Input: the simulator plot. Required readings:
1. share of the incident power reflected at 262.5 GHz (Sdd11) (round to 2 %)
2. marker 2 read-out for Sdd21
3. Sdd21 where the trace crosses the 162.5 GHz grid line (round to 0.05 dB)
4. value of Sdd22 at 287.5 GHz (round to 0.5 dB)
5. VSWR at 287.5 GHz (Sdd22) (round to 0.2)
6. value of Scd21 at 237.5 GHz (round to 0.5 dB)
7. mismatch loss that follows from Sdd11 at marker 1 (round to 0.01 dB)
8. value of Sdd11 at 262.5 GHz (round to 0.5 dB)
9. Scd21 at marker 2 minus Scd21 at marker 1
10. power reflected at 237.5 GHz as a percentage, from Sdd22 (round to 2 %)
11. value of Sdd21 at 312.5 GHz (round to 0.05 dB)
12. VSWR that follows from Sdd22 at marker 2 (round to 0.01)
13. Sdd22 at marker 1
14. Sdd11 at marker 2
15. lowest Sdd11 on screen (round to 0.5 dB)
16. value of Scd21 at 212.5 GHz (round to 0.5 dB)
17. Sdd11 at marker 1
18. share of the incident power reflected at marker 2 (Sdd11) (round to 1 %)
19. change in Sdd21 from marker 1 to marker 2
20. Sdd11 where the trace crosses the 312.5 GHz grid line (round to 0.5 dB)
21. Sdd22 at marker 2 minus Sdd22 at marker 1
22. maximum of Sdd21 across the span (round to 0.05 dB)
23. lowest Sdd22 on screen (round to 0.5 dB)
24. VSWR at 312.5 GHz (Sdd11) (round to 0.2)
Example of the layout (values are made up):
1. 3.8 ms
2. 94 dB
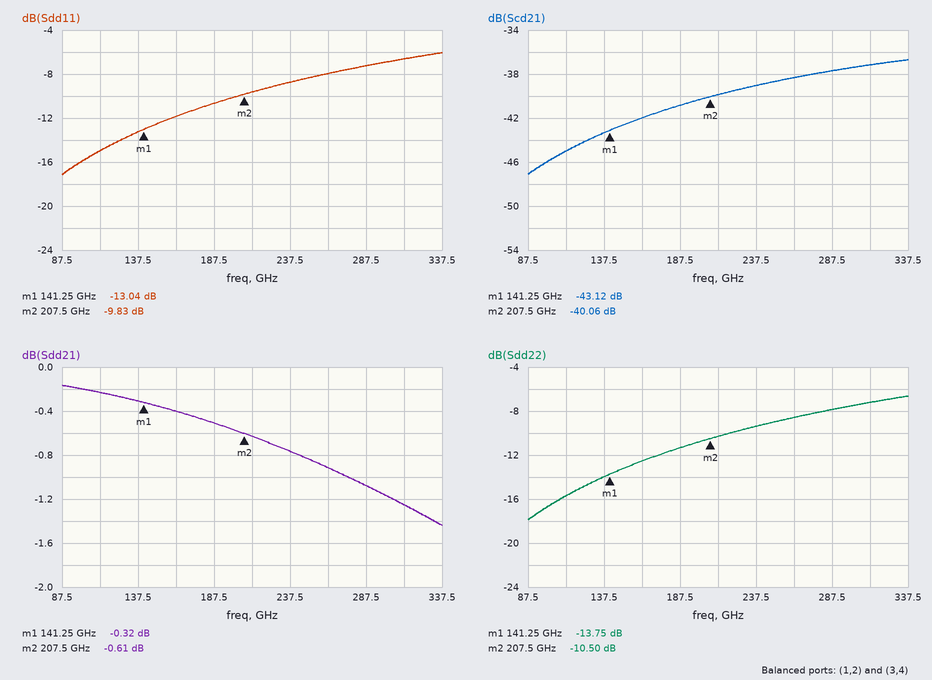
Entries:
1. 16 %
2. -0.61 dB
3. -0.40 dB
4. -8.0 dB
5. 2.4
6. -39.0 dB
7. 0.22 dB
8. -8.0 dB
9. 3.06 dB
10. 12 %
11. -1.25 dB
12. 1.85
13. -13.75 dB
14. -9.83 dB
15. -17.0 dB
16. -40.0 dB
17. -13.04 dB
18. 10 %
19. -0.29 dB
20. -6.5 dB
21. 3.25 dB
22. -0.15 dB
23. -18.0 dB
24. 2.8
